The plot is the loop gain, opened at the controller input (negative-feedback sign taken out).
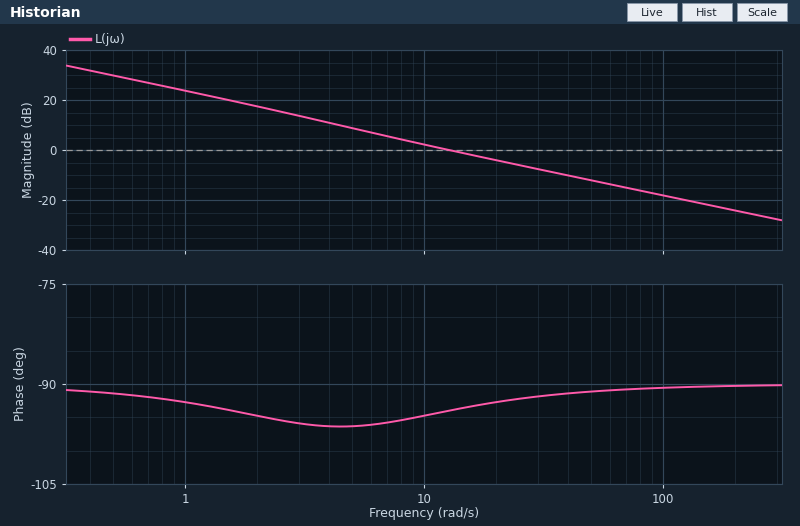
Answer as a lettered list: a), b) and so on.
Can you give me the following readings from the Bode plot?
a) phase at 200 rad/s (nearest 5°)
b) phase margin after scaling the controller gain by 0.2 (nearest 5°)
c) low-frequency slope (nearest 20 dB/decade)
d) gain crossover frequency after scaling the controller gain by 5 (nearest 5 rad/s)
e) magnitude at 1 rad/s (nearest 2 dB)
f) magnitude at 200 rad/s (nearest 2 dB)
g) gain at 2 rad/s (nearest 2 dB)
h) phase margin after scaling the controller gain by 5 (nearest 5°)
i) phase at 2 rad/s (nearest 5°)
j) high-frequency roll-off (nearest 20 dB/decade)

a) -90°
b) 85°
c) -20 dB/decade
d) 60 rad/s
e) 24 dB
f) -24 dB
g) 18 dB
h) 90°
i) -95°
j) -20 dB/decade
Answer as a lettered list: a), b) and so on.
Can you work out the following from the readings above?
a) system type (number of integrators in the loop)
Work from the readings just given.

a) 1
